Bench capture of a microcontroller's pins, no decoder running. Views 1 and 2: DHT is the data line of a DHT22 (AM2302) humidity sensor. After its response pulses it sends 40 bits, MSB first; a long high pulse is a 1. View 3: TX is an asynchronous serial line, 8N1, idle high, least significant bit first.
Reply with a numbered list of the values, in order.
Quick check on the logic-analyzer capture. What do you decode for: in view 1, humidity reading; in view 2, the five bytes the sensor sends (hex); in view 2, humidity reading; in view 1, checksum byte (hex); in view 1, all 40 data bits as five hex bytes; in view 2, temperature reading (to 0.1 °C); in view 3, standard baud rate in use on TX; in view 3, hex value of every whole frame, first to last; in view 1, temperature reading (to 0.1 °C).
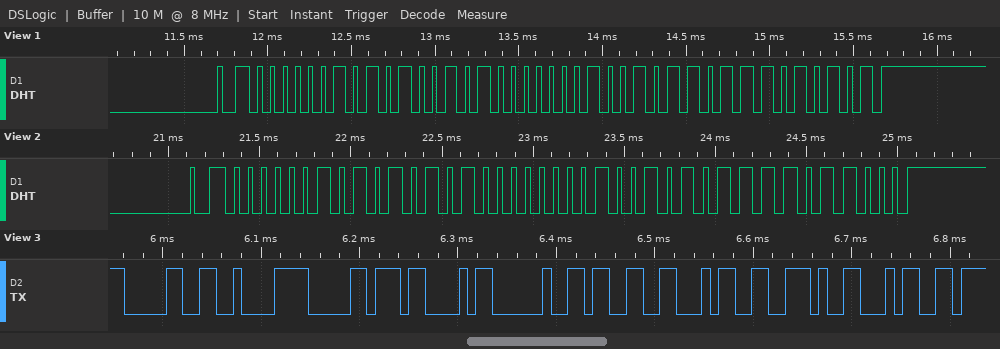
1. 67.7 %
2. 02 AA 01 2B D8
3. 68.2 %
4. 0xD5
5. 02 A5 01 2D D5
6. 29.9 °C
7. 115200 baud
8. 30 C2 B0 43 20 33 34 2E 34
9. 30.1 °C
